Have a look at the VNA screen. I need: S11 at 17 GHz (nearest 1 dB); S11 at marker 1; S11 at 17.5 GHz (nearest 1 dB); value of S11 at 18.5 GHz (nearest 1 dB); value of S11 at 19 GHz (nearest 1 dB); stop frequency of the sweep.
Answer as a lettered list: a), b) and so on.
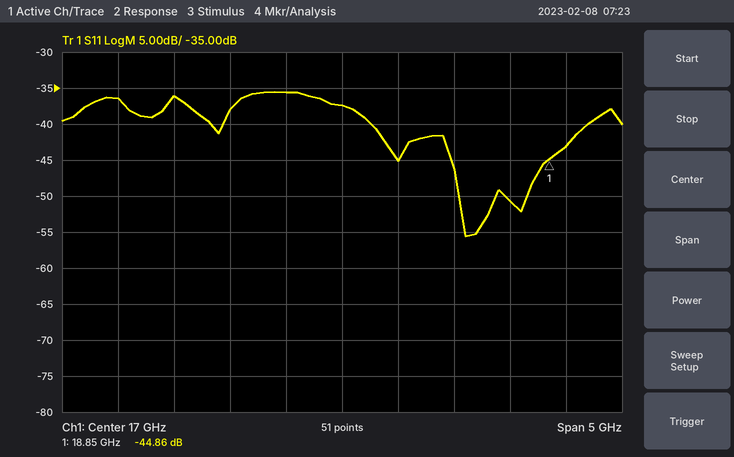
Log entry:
a) -37 dB
b) -44.86 dB
c) -45 dB
d) -51 dB
e) -43 dB
f) 19.5 GHz
